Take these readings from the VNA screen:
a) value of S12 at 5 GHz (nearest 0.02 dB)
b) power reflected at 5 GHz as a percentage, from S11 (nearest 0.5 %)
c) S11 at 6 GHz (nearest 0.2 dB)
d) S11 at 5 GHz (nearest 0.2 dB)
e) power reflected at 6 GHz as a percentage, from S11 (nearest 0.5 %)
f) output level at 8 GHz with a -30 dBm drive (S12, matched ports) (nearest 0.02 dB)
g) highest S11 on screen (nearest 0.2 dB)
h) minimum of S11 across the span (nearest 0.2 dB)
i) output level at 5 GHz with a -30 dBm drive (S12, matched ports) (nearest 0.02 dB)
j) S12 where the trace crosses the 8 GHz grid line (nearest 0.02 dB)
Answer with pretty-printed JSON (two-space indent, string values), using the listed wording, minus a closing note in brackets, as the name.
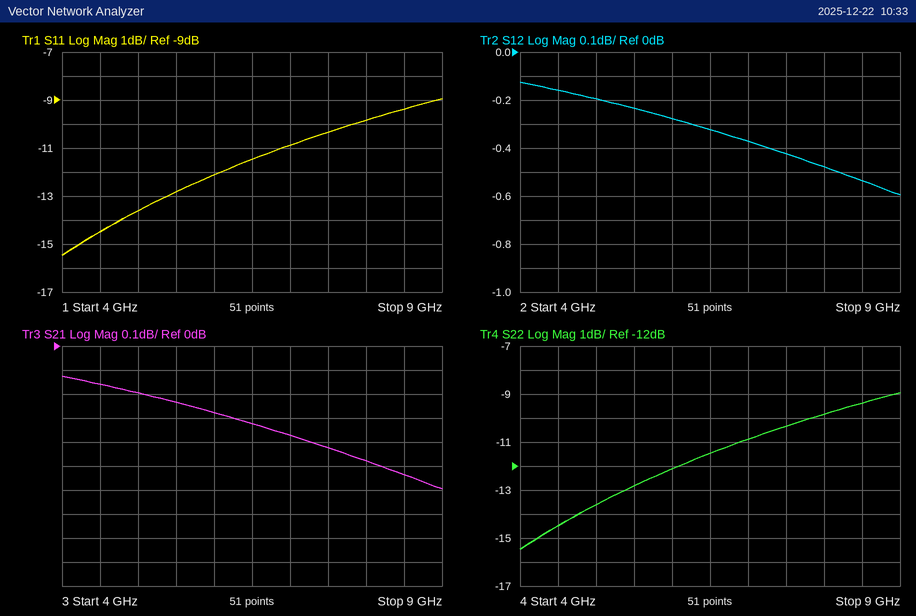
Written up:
{
  "value of S12 at 5 GHz": "-0.20 dB",
  "power reflected at 5 GHz as a percentage, from S11": "4.5 %",
  "S11 at 6 GHz": "-12.2 dB",
  "S11 at 5 GHz": "-13.6 dB",
  "power reflected at 6 GHz as a percentage, from S11": "6.0 %",
  "output level at 8 GHz with a -30 dBm drive (S12, matched ports)": "-30.48 dBm",
  "highest S11 on screen": "-9.0 dB",
  "minimum of S11 across the span": "-15.4 dB",
  "output level at 5 GHz with a -30 dBm drive (S12, matched ports)": "-30.20 dBm",
  "S12 where the trace crosses the 8 GHz grid line": "-0.48 dB"
}
